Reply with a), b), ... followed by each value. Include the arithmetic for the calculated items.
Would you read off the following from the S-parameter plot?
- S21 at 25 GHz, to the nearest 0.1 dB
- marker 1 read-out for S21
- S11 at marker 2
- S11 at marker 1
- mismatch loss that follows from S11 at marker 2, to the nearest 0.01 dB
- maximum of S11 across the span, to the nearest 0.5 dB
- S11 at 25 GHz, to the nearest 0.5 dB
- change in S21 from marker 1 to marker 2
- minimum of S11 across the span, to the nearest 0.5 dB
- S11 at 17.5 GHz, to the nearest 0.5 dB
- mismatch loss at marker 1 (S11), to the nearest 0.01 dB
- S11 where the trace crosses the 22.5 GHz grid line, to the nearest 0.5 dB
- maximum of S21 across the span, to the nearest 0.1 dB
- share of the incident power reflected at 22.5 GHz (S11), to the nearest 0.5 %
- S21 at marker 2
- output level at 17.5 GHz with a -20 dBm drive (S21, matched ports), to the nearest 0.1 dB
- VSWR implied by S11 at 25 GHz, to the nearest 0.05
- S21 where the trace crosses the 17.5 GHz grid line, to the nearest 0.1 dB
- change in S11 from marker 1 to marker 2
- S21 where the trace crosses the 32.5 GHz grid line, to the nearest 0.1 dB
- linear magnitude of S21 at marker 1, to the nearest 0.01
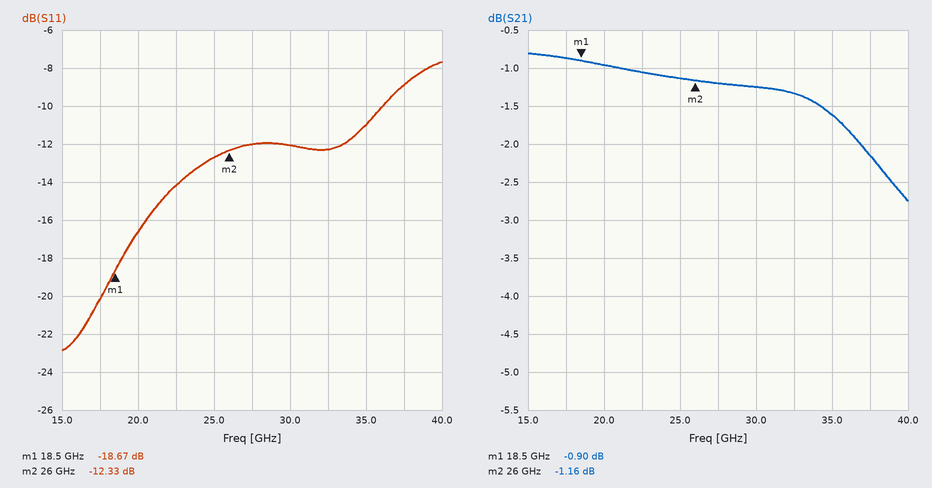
a) -1.1 dB
b) -0.90 dB
c) -12.33 dB
d) -18.67 dB
e) −10 log10(1 − 10^(-12.33/10)) ≈ 0.26 dB
f) -7.5 dB
g) -12.5 dB
h) -1.16 − (-0.9) = -0.26 dB
i) -23.0 dB
j) -20.0 dB
k) −10 log10(1 − 10^(-18.67/10)) ≈ 0.06 dB
l) -14.0 dB
m) -0.8 dB
n) 10^(-14/10) ≈ 4.0 %
o) -1.16 dB
p) -20 dBm + (-0.9 dB) = -20.9 dBm
q) |Γ| = 10^(-12.5/20) = 0.2371; VSWR = (1 + 0.2371)/(1 − 0.2371) ≈ 1.62, so 1.60 to the nearest 0.05
r) -0.9 dB
s) -12.33 − (-18.67) = 6.34 dB
t) -1.3 dB
u) 10^(-0.9/20) ≈ 0.90
